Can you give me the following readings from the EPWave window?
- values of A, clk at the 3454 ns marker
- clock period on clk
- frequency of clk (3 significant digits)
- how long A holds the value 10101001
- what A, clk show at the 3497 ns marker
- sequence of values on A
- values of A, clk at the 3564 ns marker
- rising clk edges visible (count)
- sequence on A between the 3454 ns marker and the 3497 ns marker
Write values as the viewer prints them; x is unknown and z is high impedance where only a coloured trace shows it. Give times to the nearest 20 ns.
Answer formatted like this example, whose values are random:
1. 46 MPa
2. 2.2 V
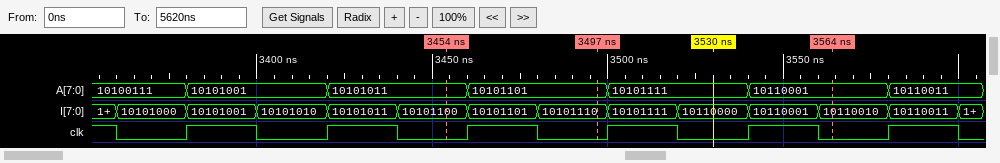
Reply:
1. A=10101011, clk=0
2. 40 ns
3. 25.0 MHz
4. 40 ns
5. A=10101101, clk=0
6. 10100111, 10101001, 10101011, 10101101, 10101111, 10110001, 10110011
7. A=10110001, clk=0
8. 6
9. 10101011, 10101101
